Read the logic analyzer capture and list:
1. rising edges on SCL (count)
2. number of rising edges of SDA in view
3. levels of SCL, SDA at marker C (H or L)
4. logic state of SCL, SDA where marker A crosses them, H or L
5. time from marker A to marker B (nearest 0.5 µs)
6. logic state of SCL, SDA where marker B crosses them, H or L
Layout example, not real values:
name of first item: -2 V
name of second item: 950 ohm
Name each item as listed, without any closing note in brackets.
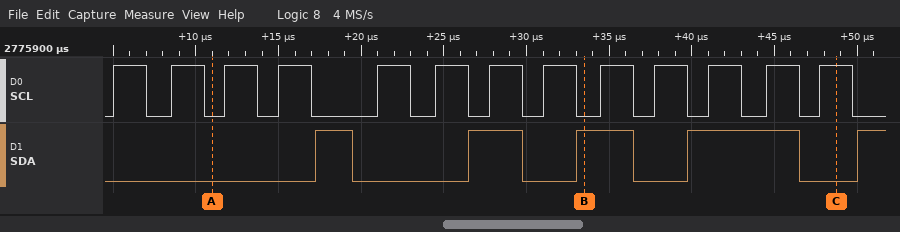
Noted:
rising edges on SCL: 13
number of rising edges of SDA in view: 5
levels of SCL, SDA at marker C: SCL=H, SDA=L
logic state of SCL, SDA where marker A crosses them, H or L: SCL=L, SDA=L
time from marker A to marker B: 22.5 µs
logic state of SCL, SDA where marker B crosses them, H or L: SCL=L, SDA=H
